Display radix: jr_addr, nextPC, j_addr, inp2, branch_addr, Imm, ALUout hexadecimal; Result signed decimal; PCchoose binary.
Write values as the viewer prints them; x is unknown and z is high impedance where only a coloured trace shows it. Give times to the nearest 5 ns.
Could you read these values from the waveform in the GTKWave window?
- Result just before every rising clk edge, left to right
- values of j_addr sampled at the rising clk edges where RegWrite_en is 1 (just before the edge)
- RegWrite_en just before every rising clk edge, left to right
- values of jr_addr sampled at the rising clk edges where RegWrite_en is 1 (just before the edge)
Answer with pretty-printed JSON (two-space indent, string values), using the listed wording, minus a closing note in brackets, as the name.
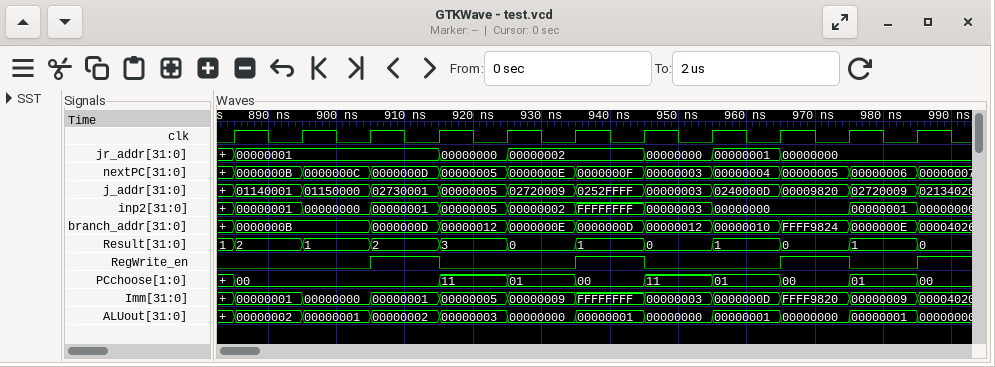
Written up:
{
  "Result just before every rising clk edge, left to right": "1, 2, 1, 2, 3, 0, 1, 0, 1, 0, 1",
  "values of j_addr sampled at the rising clk edges where RegWrite_en is 1": "02730001, 0252FFFF, 00009820",
  "RegWrite_en just before every rising clk edge, left to right": "0 0 0 1 0 0 1 0 0 1 0",
  "values of jr_addr sampled at the rising clk edges where RegWrite_en is 1": "00000001, 00000002, 00000000"
}
